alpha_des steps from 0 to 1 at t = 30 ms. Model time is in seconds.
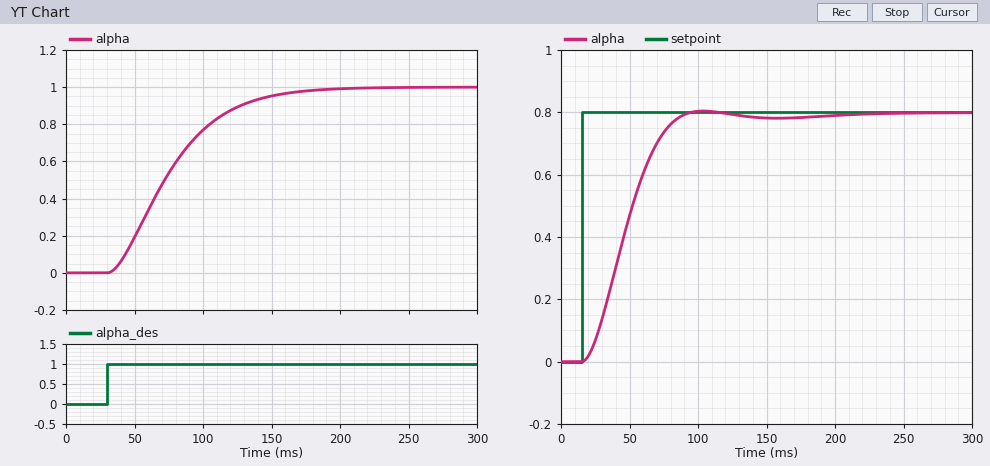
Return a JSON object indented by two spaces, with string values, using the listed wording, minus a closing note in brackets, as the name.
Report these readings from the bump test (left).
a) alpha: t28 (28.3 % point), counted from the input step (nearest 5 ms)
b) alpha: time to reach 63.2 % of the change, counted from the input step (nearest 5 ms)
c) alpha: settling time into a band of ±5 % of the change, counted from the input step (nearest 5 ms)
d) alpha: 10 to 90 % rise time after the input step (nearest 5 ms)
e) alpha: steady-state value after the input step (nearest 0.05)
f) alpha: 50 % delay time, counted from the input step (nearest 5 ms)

{
  "alpha: t28 (28.3 % point), counted from the input step": "25 ms",
  "alpha: time to reach 63.2 % of the change, counted from the input step": "55 ms",
  "alpha: settling time into a band of ±5 % of the change, counted from the input step": "120 ms",
  "alpha: 10 to 90 % rise time after the input step": "85 ms",
  "alpha: steady-state value after the input step": "1.00",
  "alpha: 50 % delay time, counted from the input step": "40 ms"
}
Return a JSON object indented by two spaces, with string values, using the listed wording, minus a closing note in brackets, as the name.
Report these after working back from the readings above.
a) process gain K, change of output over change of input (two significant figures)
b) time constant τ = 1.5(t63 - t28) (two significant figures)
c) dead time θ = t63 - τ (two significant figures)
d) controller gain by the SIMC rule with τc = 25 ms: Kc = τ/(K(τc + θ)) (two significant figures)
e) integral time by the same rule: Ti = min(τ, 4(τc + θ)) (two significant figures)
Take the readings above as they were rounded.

{
  "process gain K, change of output over change of input": "1.0",
  "time constant τ = 1.5(t63 - t28)": "45 ms",
  "dead time θ = t63 - τ": "10 ms",
  "controller gain by the SIMC rule with τc = 25 ms: Kc = τ/(K(τc + θ))": "1.3",
  "integral time by the same rule: Ti = min(τ, 4(τc + θ))": "45 ms"
}
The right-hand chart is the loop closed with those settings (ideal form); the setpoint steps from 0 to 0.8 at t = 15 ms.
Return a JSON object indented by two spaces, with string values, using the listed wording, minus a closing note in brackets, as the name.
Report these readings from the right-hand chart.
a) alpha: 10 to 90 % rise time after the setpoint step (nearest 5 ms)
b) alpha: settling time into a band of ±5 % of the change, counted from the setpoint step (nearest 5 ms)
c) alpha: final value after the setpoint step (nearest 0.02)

{
  "alpha: 10 to 90 % rise time after the setpoint step": "45 ms",
  "alpha: settling time into a band of ±5 % of the change, counted from the setpoint step": "65 ms",
  "alpha: final value after the setpoint step": "0.80"
}
